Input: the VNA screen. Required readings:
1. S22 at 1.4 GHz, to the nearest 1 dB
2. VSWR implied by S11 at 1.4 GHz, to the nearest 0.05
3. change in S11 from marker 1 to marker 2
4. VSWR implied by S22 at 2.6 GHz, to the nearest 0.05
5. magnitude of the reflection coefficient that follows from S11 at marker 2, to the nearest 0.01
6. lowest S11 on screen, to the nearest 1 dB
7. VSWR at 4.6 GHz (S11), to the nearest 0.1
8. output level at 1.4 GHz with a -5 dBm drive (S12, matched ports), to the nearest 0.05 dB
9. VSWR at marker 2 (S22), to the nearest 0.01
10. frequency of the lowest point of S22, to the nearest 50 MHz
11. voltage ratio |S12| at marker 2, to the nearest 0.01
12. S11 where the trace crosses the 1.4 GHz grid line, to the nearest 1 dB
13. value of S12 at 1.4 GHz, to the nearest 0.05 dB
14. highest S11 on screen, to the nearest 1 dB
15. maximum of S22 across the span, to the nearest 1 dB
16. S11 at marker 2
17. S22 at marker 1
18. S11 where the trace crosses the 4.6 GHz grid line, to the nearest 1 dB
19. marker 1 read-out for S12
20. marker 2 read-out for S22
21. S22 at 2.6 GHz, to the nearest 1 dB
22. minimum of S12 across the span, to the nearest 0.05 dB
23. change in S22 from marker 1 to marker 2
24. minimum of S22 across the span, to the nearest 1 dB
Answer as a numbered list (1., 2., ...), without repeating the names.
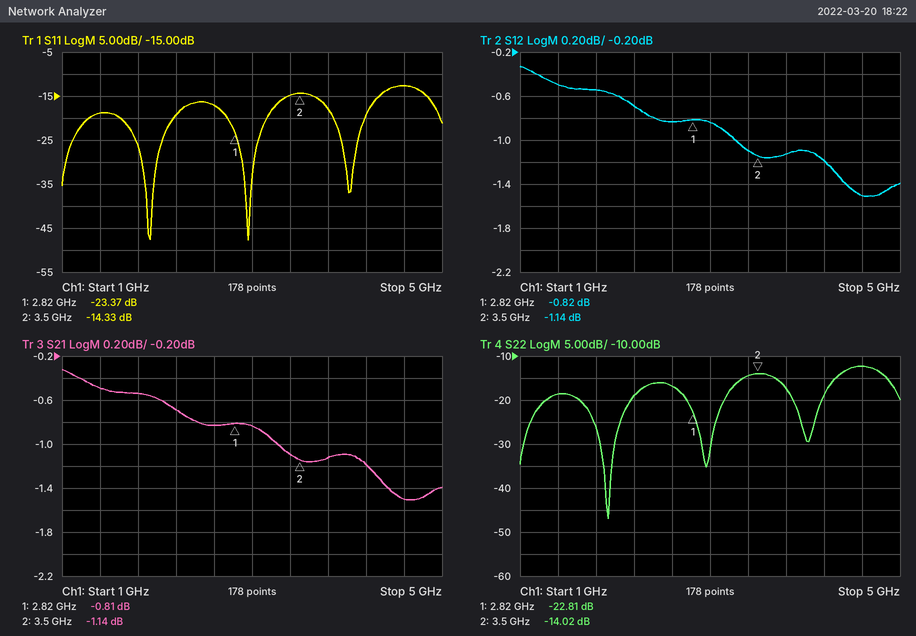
1. -19 dB
2. 1.25
3. 9.04 dB
4. 1.35
5. 0.19
6. -48 dB
7. 1.6
8. -5.50 dBm
9. 1.50
10. 1.95 GHz
11. 0.88
12. -19 dB
13. -0.50 dB
14. -13 dB
15. -12 dB
16. -14.33 dB
17. -22.81 dB
18. -13 dB
19. -0.82 dB
20. -14.02 dB
21. -17 dB
22. -1.50 dB
23. 8.79 dB
24. -47 dB
